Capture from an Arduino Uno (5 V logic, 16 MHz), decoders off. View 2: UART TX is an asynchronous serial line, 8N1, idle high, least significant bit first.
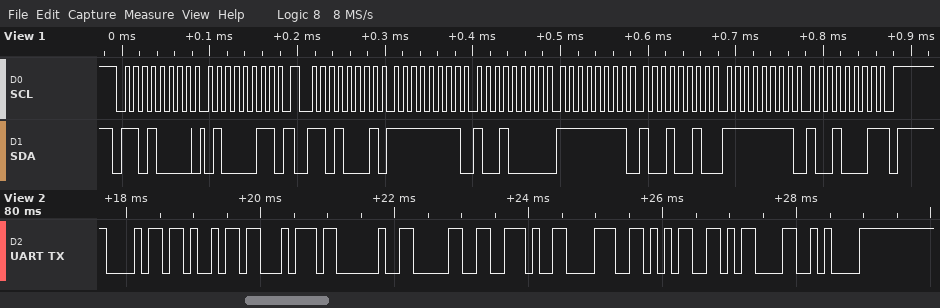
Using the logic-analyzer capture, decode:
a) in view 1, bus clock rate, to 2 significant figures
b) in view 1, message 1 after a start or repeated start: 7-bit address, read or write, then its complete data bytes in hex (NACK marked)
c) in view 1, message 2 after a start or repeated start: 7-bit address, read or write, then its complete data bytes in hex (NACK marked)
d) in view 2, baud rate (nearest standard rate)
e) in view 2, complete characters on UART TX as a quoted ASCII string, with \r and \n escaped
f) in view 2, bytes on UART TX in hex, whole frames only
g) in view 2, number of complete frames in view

100 kHz
0x68 write: 43
0x68 read: FF 90 FF 92 FF 91 NACK
9600 baud
"hit 0.85\r\n"
68 69 74 20 30 2E 38 35 0D 0A
10
